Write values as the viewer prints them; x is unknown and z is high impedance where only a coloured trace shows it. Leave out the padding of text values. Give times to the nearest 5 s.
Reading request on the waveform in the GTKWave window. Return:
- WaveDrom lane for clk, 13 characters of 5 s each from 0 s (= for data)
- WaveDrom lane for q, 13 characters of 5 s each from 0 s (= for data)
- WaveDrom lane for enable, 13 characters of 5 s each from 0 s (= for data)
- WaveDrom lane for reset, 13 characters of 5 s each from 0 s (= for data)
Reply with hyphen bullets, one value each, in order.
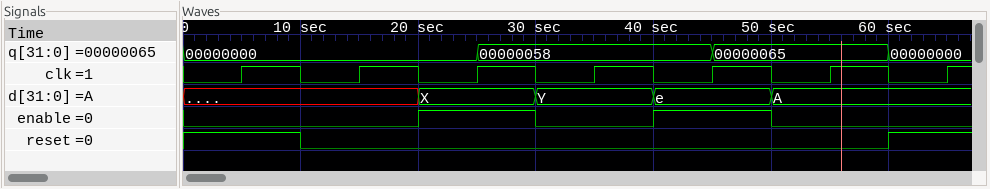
- {name: 'clk', wave: '0101010101010'}
- {name: 'q', wave: '=....=...=..=', data: '00000000 00000058 00000065 00000000'}
- {name: 'enable', wave: '0...1.0.1.0..'}
- {name: 'reset', wave: '1.0.........1'}
